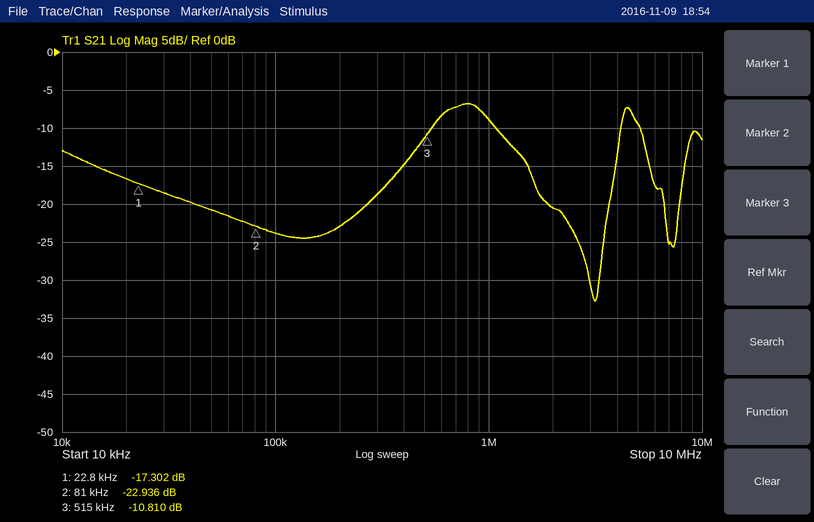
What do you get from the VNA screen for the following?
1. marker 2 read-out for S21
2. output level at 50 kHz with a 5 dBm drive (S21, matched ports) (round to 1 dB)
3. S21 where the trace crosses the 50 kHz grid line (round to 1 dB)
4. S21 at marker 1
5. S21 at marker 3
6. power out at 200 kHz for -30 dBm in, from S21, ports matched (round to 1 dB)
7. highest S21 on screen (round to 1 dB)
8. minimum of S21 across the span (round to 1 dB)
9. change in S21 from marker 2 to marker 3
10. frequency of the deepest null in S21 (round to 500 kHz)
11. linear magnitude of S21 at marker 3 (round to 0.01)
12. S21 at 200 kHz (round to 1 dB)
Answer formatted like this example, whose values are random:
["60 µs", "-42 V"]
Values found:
["-22.936 dB", "-16 dBm", "-21 dB", "-17.302 dB", "-10.810 dB", "-53 dBm", "-7 dB", "-33 dB", "12.126 dB", "3.0 MHz", "0.29", "-23 dB"]
